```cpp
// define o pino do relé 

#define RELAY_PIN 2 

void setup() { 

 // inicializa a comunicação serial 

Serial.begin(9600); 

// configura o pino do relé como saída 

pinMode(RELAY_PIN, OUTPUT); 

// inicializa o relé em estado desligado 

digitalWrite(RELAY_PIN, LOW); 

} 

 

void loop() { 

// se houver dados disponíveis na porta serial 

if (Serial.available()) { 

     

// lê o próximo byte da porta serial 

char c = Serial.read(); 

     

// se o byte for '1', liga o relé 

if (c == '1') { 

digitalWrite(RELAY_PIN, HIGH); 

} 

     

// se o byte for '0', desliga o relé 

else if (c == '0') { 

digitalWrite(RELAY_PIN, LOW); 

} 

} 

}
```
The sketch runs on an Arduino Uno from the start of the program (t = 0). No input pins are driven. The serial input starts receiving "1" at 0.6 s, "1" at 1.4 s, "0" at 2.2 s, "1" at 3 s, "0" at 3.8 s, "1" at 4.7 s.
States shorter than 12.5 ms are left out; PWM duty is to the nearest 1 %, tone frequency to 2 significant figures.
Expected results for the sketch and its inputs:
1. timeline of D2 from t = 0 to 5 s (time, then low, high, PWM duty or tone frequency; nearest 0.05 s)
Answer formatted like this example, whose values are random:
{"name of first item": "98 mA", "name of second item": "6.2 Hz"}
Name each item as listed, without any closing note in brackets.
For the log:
{"timeline of D2 from t = 0 to 5 s": "0 s low; 0.6 s high; 2.2 s low; 3 s high; 3.8 s low; 4.7 s high"}
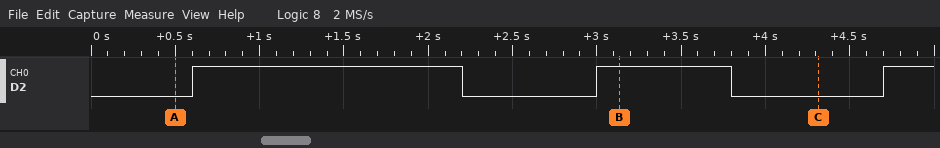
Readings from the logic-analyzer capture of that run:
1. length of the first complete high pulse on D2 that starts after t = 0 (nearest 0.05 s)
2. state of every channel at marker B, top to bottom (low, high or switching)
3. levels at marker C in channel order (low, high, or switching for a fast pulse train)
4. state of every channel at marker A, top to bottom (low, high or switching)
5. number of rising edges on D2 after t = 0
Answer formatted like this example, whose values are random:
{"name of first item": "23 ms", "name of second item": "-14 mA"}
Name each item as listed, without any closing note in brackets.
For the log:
{"length of the first complete high pulse on D2 that starts after t = 0": "1.60 s", "state of every channel at marker B, top to bottom": "D2 high", "levels at marker C in channel order": "D2 low", "state of every channel at marker A, top to bottom": "D2 low", "number of rising edges on D2 after t = 0": "3"}
